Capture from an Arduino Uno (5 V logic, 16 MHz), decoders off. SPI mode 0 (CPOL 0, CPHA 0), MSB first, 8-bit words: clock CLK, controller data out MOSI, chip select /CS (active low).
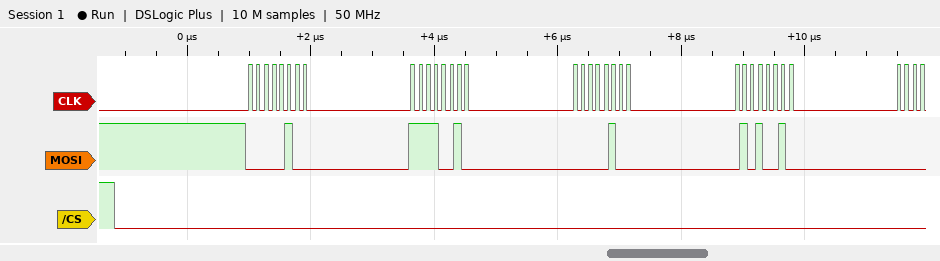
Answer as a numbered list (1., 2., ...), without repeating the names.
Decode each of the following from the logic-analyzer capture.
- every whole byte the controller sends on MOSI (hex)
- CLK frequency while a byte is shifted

1. 04 F2 04 52
2. 8 MHz
